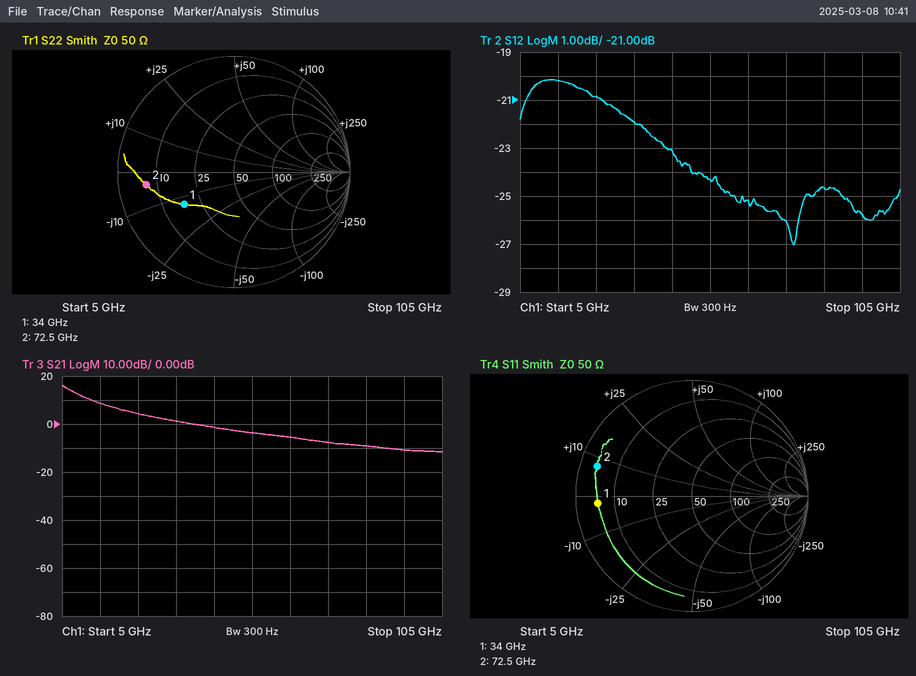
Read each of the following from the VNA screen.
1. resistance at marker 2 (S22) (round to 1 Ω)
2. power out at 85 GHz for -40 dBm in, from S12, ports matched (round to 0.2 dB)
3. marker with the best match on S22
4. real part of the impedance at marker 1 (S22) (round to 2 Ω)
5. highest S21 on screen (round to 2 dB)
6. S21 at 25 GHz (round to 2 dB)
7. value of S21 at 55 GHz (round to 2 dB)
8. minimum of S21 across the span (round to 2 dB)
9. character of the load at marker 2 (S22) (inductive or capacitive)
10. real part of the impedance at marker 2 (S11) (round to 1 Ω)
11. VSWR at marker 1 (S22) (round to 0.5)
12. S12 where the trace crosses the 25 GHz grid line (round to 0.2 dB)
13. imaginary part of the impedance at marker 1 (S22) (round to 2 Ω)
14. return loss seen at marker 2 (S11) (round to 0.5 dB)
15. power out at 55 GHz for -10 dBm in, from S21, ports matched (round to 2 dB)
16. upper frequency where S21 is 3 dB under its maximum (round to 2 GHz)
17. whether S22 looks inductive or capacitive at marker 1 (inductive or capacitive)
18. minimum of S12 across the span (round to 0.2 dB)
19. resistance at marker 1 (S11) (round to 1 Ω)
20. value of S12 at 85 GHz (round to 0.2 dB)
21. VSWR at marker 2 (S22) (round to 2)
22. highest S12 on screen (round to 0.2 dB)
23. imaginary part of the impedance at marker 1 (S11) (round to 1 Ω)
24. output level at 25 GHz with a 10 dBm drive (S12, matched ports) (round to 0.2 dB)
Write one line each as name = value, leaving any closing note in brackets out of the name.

resistance at marker 2 (S22) = 7 Ω
power out at 85 GHz for -40 dBm in, from S12, ports matched = -64.6 dBm
marker with the best match on S22 = marker 1
real part of the impedance at marker 1 (S22) = 18 Ω
highest S21 on screen = 16 dB
S21 at 25 GHz = 4 dB
value of S21 at 55 GHz = -4 dB
minimum of S21 across the span = -12 dB
character of the load at marker 2 (S22) = capacitive
real part of the impedance at marker 2 (S11) = 4 Ω
VSWR at marker 1 (S22) = 3.0
S12 where the trace crosses the 25 GHz grid line = -20.8 dB
imaginary part of the impedance at marker 1 (S22) = -14 Ω
return loss seen at marker 2 (S11) = 1.5 dB
power out at 55 GHz for -10 dBm in, from S21, ports matched = -14 dBm
upper frequency where S21 is 3 dB under its maximum = 8 GHz
whether S22 looks inductive or capacitive at marker 1 = capacitive
minimum of S12 across the span = -27.0 dB
resistance at marker 1 (S11) = 5 Ω
value of S12 at 85 GHz = -24.6 dB
VSWR at marker 2 (S22) = 8
highest S12 on screen = -20.2 dB
imaginary part of the impedance at marker 1 (S11) = -2 Ω
output level at 25 GHz with a 10 dBm drive (S12, matched ports) = -10.8 dBm
